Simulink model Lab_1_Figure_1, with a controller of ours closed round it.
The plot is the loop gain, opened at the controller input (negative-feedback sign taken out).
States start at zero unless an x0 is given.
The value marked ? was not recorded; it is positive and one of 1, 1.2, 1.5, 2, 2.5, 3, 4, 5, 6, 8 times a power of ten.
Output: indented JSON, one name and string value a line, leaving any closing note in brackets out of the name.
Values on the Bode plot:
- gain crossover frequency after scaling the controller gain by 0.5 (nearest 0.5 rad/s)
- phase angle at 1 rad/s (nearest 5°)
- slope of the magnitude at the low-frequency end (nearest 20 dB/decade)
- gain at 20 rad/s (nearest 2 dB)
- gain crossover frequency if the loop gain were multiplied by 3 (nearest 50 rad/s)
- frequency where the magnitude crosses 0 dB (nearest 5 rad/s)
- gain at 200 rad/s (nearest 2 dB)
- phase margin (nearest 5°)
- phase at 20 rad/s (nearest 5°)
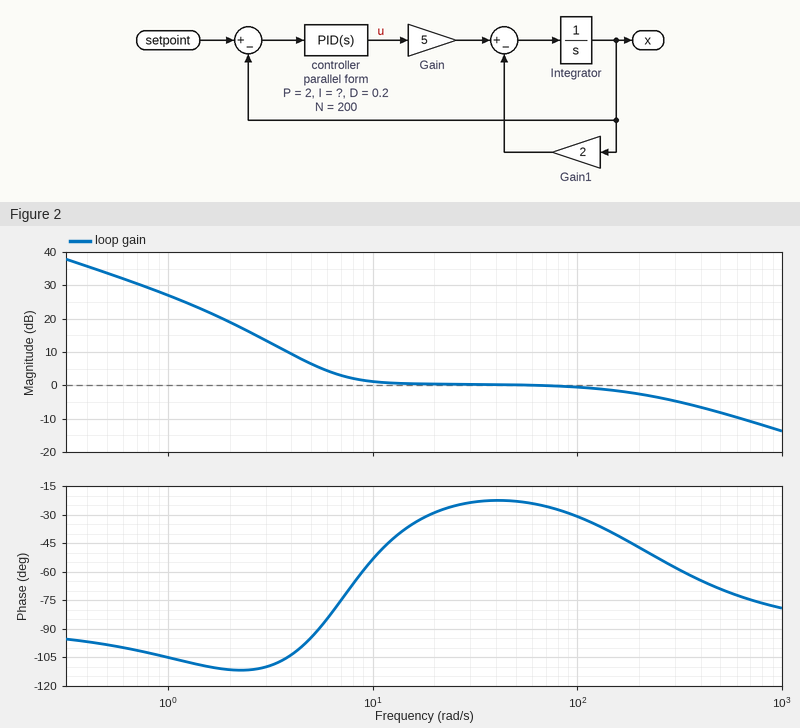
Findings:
{
  "gain crossover frequency after scaling the controller gain by 0.5": "5.0 rad/s",
  "phase angle at 1 rad/s": "-105°",
  "slope of the magnitude at the low-frequency end": "-20 dB/decade",
  "gain at 20 rad/s": "0 dB",
  "gain crossover frequency if the loop gain were multiplied by 3": "600 rad/s",
  "frequency where the magnitude crosses 0 dB": "65 rad/s",
  "gain at 200 rad/s": "-2 dB",
  "phase margin": "155°",
  "phase at 20 rad/s": "-30°"
}
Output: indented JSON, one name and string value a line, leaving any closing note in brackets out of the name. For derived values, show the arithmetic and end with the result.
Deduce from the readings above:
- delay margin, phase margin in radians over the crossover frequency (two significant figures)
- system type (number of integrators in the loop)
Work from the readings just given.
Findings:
{
  "delay margin, phase margin in radians over the crossover frequency": "155 × π / 180 / 65 = 0.042 s",
  "system type": "1"
}
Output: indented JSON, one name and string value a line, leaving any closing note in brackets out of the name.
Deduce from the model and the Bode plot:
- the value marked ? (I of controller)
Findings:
{
  "the value marked ?": "10"
}
